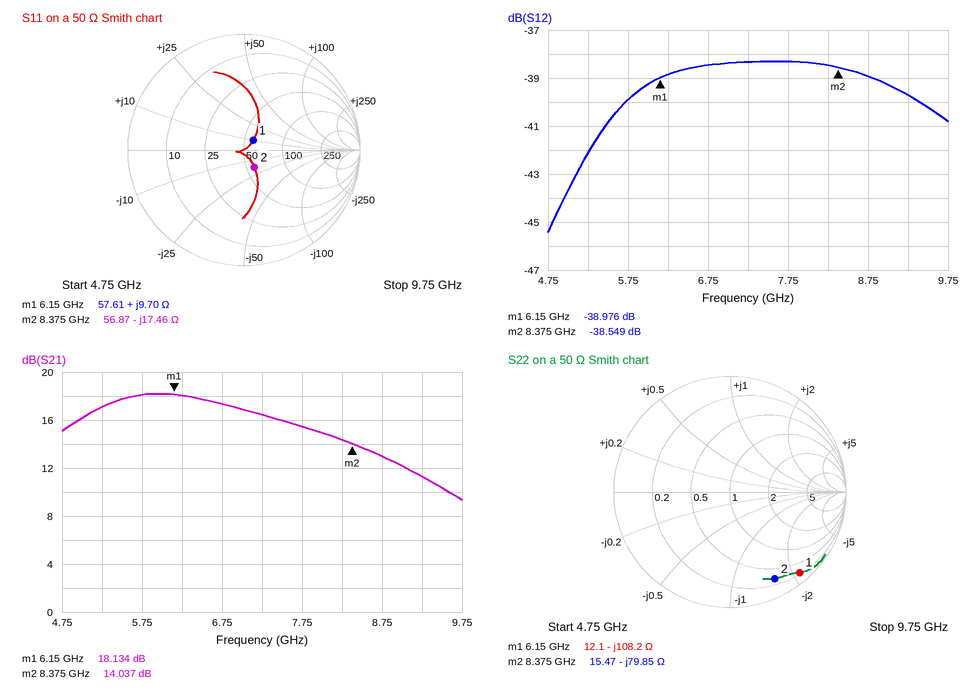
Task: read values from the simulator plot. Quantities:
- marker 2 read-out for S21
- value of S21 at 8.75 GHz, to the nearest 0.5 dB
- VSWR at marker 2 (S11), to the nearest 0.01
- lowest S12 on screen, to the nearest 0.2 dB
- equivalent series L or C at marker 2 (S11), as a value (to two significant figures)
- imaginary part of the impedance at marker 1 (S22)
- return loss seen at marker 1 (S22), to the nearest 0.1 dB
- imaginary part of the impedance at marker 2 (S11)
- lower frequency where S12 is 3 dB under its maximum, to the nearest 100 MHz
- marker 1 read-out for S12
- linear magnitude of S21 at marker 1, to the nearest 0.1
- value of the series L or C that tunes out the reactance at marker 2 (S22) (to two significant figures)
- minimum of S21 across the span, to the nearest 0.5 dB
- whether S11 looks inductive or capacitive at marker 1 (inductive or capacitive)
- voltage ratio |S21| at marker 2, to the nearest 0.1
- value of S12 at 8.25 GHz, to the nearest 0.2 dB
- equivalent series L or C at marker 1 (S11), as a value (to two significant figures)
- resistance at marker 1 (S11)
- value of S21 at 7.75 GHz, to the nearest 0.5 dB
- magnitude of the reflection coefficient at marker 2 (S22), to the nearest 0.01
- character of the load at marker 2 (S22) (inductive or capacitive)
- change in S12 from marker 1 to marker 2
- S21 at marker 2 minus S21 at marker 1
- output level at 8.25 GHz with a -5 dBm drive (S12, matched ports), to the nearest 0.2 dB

14.037 dB
13.0 dB
1.42
-45.4 dB
1.1 pF
-108.2 Ω
0.7 dB
-17.46 Ω
5.4 GHz
-38.976 dB
8.1
1.5 nH
9.5 dB
inductive
5.0
-38.4 dB
250 pH
57.61 Ω
15.5 dB
0.84
capacitive
0.427 dB
-4.097 dB
-43.4 dBm
